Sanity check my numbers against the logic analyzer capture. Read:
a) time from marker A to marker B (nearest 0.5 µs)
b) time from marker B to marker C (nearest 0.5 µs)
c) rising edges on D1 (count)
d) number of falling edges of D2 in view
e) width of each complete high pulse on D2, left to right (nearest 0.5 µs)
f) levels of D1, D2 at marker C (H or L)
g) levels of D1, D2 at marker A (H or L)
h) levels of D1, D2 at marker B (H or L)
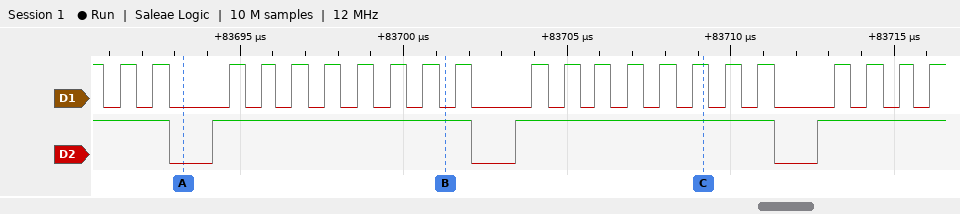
8 µs
8 µs
22
3
8 µs, 8 µs
D1=H, D2=H
D1=L, D2=L
D1=L, D2=H
